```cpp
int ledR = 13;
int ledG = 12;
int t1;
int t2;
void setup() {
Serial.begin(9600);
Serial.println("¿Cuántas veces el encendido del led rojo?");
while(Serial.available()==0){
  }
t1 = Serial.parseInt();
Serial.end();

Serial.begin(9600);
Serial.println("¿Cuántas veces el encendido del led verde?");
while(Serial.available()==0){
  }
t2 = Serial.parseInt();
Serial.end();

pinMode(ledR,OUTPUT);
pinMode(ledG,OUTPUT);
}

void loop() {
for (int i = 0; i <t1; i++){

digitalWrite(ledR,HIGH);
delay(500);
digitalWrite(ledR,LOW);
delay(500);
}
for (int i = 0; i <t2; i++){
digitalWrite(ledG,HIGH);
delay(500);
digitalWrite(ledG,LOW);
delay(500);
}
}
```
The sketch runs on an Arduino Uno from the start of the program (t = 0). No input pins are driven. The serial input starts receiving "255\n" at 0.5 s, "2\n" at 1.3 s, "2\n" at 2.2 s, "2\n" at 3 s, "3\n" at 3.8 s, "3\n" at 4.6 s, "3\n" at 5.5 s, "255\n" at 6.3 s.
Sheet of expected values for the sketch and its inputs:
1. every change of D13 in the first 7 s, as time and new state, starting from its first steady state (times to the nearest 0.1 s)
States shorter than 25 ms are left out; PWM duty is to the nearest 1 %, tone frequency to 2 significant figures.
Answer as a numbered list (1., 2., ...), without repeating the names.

1. 1.3 s high; 1.8 s low; 2.3 s high; 2.8 s low; 3.3 s high; 3.8 s low; 4.3 s high; 4.8 s low; 5.3 s high; 5.8 s low; 6.3 s high; 6.8 s low
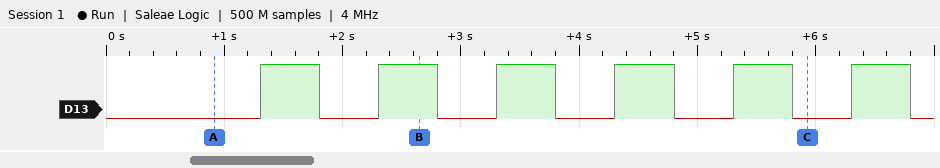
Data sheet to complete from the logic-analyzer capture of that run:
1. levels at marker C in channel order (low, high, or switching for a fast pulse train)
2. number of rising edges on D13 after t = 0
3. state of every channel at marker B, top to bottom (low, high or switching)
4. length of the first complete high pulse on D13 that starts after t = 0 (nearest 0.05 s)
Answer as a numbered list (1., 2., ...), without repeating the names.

1. D13 low
2. 6
3. D13 high
4. 0.50 s
